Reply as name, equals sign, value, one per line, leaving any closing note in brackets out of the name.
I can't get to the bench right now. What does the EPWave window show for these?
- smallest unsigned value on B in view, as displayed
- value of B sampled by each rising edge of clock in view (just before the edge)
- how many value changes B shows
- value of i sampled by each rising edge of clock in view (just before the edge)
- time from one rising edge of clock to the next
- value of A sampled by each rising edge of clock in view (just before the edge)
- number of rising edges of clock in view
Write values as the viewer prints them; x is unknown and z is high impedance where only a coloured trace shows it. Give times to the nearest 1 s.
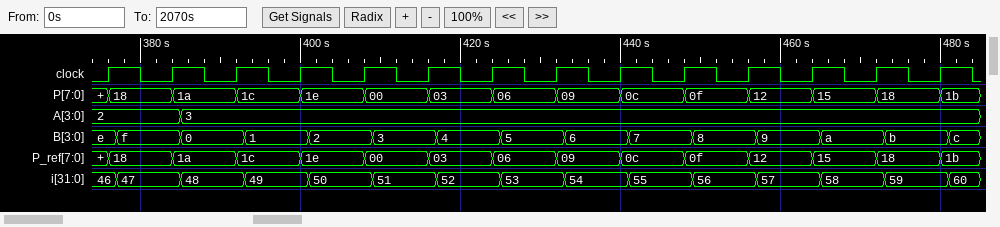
smallest unsigned value on B in view, as displayed = 0
value of B sampled by each rising edge of clock in view = e, f, 0, 1, 2, 3, 4, 5, 6, 7, 8, 9, a, b
how many value changes B shows = 14
value of i sampled by each rising edge of clock in view = 46, 47, 48, 49, 50, 51, 52, 53, 54, 55, 56, 57, 58, 59
time from one rising edge of clock to the next = 8 s
value of A sampled by each rising edge of clock in view = 2, 2, 3, 3, 3, 3, 3, 3, 3, 3, 3, 3, 3, 3
number of rising edges of clock in view = 14
